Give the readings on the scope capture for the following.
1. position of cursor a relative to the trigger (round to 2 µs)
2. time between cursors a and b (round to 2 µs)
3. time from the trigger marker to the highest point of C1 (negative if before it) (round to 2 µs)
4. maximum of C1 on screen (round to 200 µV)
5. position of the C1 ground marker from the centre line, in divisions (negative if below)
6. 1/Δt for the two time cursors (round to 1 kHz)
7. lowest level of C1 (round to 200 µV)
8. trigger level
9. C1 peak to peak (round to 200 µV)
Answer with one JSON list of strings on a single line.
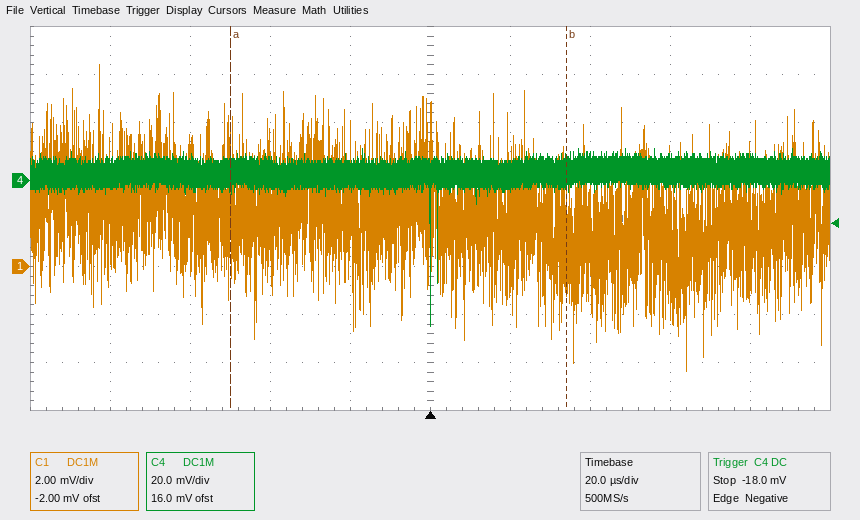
["-50 µs", "84 µs", "-82 µs", "8.4 mV", "-1.0 div", "12 kHz", "-4.4 mV", "-18.0 mV", "12.8 mV"]
